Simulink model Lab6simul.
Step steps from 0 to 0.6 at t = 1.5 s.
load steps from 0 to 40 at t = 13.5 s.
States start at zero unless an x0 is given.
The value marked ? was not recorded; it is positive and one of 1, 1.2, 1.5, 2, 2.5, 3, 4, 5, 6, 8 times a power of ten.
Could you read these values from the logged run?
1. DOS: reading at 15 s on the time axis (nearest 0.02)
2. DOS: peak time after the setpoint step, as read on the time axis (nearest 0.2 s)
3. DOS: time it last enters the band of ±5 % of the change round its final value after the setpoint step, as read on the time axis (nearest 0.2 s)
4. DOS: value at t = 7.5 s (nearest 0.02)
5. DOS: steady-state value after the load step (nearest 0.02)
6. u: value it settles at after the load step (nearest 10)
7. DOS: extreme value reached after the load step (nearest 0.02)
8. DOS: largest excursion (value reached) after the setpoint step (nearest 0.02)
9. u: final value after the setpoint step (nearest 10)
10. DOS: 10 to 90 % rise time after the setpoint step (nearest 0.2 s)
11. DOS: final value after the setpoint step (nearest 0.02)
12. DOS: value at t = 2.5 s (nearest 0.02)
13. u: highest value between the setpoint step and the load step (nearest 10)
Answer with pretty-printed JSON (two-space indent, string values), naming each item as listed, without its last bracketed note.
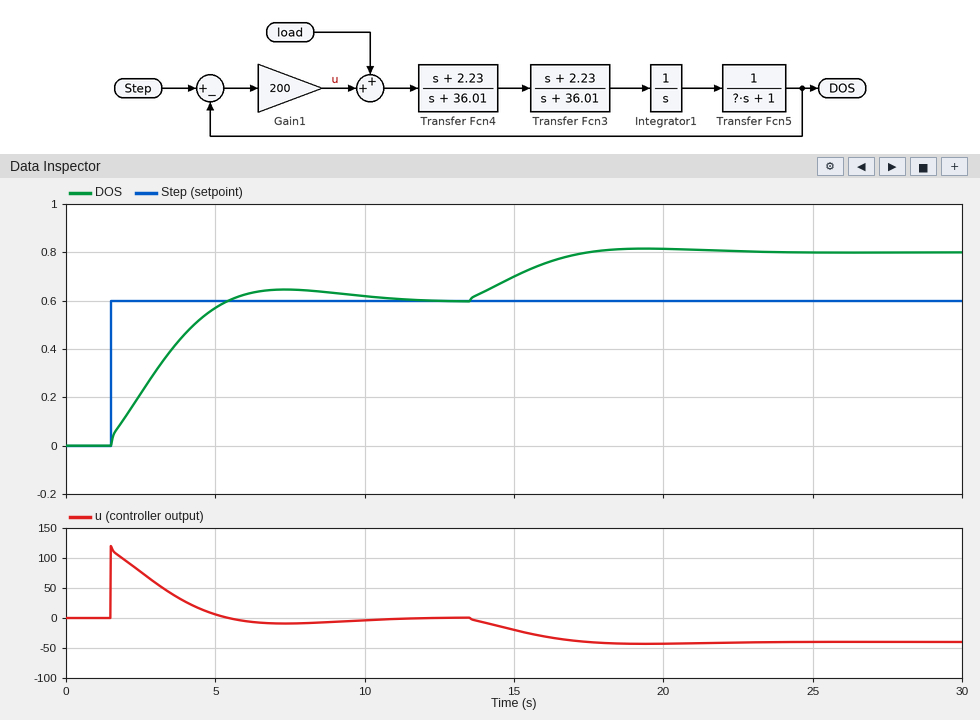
{
  "DOS: reading at 15 s on the time axis": "0.70",
  "DOS: peak time after the setpoint step, as read on the time axis": "7.4 s",
  "DOS: time it last enters the band of ±5 % of the change round its final value after the setpoint step, as read on the time axis": "9.2 s",
  "DOS: value at t = 7.5 s": "0.64",
  "DOS: steady-state value after the load step": "0.80",
  "u: value it settles at after the load step": "-40",
  "DOS: extreme value reached after the load step": "0.82",
  "DOS: largest excursion (value reached) after the setpoint step": "0.64",
  "u: final value after the setpoint step": "0",
  "DOS: 10 to 90 % rise time after the setpoint step": "3.0 s",
  "DOS: final value after the setpoint step": "0.60",
  "DOS: value at t = 2.5 s": "0.22",
  "u: highest value between the setpoint step and the load step": "120"
}
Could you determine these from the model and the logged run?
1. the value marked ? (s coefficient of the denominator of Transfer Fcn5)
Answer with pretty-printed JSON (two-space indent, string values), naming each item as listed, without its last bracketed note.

{
  "the value marked ?": "2"
}
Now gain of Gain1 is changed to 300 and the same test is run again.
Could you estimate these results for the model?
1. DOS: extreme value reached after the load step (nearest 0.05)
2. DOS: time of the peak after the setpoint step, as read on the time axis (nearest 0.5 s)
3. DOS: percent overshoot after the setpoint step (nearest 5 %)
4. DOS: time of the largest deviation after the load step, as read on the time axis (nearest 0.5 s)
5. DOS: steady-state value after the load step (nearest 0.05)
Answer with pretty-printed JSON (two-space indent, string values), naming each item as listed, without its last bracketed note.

{
  "DOS: extreme value reached after the load step": "0.75",
  "DOS: time of the peak after the setpoint step, as read on the time axis": "6.0 s",
  "DOS: percent overshoot after the setpoint step": "10 %",
  "DOS: time of the largest deviation after the load step, as read on the time axis": "18.0 s",
  "DOS: steady-state value after the load step": "0.75"
}
